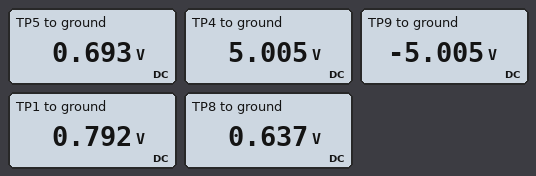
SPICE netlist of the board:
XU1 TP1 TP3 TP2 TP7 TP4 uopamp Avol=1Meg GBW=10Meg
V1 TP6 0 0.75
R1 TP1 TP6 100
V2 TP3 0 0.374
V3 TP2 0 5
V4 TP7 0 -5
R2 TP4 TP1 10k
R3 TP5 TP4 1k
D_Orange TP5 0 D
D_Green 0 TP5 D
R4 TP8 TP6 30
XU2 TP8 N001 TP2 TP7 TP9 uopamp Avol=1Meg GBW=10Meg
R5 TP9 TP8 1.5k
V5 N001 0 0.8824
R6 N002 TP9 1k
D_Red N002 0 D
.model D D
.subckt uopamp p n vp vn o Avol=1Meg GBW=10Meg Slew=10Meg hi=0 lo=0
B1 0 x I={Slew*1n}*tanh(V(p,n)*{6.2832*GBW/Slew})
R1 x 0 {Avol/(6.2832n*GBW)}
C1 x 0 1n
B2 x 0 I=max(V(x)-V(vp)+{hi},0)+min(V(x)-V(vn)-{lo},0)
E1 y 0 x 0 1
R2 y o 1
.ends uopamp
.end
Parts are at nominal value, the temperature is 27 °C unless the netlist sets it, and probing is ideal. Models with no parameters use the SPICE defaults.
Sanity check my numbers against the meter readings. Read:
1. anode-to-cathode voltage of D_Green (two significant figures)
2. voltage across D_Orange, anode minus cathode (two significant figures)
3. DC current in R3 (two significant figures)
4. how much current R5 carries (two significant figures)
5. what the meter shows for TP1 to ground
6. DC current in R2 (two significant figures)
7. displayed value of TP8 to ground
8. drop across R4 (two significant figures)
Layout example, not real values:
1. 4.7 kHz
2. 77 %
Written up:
1. -690 mV
2. 690 mV
3. 4.3 mA
4. 3.8 mA
5. 0.792 V
6. 420 µA
7. 0.637 V
8. 110 mV
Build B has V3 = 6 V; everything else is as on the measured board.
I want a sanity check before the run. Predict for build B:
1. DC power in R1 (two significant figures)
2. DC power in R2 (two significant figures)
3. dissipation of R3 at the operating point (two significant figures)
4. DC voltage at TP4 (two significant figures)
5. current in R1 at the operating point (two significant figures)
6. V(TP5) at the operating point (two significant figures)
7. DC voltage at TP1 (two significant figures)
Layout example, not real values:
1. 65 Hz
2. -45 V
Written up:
1. 27 µW
2. 2.7 mW
3. 28 mW
4. 6.0 V
5. 520 µA
6. 700 mV
7. 800 mV
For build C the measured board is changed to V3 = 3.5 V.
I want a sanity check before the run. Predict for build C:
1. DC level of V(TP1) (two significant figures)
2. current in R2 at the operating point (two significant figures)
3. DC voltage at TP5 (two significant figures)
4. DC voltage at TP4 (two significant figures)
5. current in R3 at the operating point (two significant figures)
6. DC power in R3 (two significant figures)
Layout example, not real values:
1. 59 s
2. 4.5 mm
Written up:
1. 780 mV
2. 270 µA
3. 680 mV
4. 3.5 V
5. 2.8 mA
6. 8.0 mW
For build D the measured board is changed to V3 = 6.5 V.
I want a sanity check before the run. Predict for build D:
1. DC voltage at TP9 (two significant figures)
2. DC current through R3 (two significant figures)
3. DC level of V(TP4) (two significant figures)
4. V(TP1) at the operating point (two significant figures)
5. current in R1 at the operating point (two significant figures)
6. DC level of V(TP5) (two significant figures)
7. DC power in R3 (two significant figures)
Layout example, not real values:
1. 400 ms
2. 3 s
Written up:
1. -5.0 V
2. 5.8 mA
3. 6.5 V
4. 810 mV
5. 570 µA
6. 700 mV
7. 34 mW
